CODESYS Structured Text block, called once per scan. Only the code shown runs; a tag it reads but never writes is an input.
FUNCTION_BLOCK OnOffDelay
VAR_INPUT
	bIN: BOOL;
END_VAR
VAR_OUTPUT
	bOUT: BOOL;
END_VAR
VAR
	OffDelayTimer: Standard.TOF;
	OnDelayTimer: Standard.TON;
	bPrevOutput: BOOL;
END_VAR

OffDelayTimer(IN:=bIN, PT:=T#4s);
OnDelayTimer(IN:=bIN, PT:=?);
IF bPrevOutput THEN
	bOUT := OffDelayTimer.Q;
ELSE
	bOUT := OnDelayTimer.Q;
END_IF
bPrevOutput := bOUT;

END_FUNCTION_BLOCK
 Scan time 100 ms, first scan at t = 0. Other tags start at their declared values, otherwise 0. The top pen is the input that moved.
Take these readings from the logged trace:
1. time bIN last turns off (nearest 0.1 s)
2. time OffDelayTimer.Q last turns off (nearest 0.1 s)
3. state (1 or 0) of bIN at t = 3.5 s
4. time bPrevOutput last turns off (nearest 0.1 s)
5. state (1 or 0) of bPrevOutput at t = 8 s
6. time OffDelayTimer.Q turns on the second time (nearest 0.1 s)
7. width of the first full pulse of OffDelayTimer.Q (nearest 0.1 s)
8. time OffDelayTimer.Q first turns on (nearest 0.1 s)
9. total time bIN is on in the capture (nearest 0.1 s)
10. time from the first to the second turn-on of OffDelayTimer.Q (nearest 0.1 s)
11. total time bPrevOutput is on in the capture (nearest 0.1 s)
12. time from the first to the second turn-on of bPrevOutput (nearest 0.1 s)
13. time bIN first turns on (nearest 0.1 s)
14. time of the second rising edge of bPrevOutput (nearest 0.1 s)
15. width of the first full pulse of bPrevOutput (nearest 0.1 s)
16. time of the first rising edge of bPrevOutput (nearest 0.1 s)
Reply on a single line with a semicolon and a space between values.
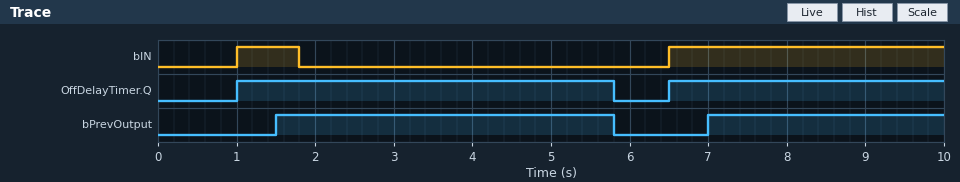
1.8 s; 5.8 s; 0; 5.8 s; 1; 6.5 s; 4.8 s; 1.0 s; 4.3 s; 5.5 s; 7.3 s; 5.5 s; 1.0 s; 7.0 s; 4.3 s; 1.5 s
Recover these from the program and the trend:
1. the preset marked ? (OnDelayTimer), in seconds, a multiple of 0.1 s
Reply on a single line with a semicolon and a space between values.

0.5 s
